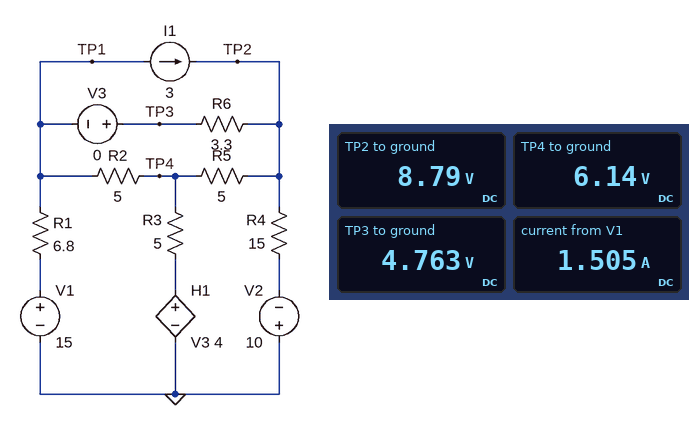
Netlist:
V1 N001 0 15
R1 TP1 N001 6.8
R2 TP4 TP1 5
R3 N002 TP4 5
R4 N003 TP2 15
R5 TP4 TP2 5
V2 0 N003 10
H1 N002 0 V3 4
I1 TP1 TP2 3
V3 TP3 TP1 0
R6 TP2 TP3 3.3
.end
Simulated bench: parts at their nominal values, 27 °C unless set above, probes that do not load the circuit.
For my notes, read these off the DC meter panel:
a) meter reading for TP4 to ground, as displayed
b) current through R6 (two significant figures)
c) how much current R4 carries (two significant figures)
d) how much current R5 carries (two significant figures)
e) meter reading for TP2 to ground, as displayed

6.14 V
1.2 A
1.3 A
530 mA
8.79 V
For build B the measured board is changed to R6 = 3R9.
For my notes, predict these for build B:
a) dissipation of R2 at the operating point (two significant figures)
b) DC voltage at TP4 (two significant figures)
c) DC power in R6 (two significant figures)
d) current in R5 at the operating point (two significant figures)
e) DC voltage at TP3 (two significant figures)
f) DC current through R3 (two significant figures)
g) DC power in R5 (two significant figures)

470 mW
6.0 V
5.1 W
590 mA
4.5 V
280 mA
1.7 W
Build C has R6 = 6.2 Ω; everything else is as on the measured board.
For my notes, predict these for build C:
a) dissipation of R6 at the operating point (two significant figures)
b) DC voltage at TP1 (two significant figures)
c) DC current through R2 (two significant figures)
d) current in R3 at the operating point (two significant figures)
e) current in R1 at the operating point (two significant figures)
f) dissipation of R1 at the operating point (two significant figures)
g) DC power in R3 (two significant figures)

5.4 W
3.6 V
390 mA
370 mA
1.7 A
19 W
700 mW
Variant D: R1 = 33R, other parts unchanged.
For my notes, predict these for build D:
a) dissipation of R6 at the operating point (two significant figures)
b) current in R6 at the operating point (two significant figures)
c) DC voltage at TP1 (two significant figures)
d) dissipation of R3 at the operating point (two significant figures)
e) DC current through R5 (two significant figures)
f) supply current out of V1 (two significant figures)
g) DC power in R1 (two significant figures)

9.5 W
1.7 A
-230 mV
1.6 W
280 mA
460 mA
7.0 W
